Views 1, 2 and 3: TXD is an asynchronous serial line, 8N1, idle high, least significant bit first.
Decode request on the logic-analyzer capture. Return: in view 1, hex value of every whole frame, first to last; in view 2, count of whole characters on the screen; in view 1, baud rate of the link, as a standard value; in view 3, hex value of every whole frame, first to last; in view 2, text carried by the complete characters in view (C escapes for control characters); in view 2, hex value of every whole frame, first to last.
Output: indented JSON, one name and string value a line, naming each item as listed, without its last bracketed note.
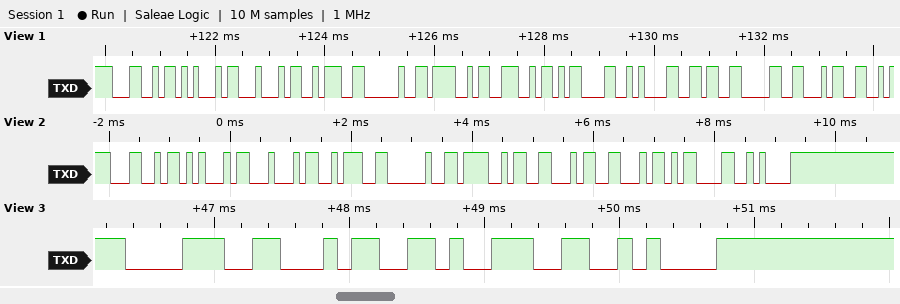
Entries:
{
  "in view 1, hex value of every whole frame, first to last": "4C 45 44 3A 20 4F 4E 0D 0A 36 30 34",
  "in view 2, count of whole characters on the screen": "10",
  "in view 1, baud rate of the link, as a standard value": "9600 baud",
  "in view 3, hex value of every whole frame, first to last": "38 34 39 0A",
  "in view 2, text carried by the complete characters in view": "\"LED: OFF\\r\\n\"",
  "in view 2, hex value of every whole frame, first to last": "4C 45 44 3A 20 4F 46 46 0D 0A"
}
